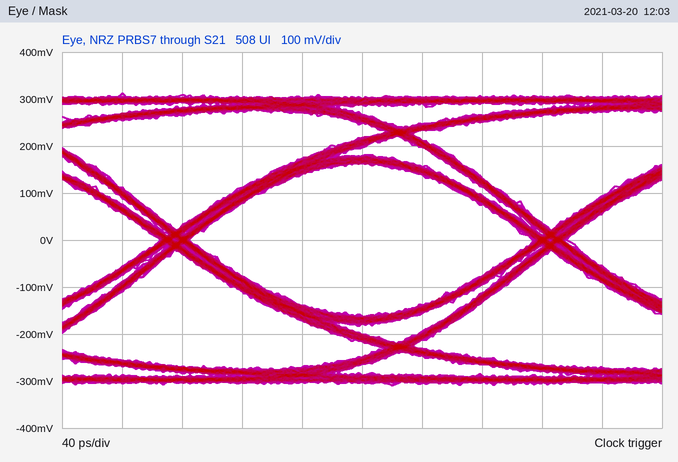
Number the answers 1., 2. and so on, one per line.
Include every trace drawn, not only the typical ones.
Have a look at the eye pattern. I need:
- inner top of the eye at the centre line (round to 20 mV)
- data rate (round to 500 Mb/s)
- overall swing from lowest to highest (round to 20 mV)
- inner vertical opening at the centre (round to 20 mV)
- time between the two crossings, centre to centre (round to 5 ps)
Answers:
1. 160 mV
2. 4.0 Gb/s
3. 620 mV
4. 320 mV
5. 250 ps
